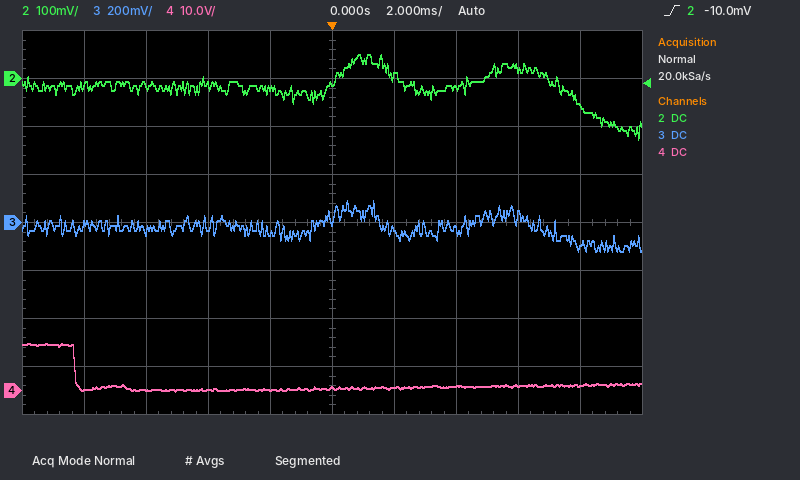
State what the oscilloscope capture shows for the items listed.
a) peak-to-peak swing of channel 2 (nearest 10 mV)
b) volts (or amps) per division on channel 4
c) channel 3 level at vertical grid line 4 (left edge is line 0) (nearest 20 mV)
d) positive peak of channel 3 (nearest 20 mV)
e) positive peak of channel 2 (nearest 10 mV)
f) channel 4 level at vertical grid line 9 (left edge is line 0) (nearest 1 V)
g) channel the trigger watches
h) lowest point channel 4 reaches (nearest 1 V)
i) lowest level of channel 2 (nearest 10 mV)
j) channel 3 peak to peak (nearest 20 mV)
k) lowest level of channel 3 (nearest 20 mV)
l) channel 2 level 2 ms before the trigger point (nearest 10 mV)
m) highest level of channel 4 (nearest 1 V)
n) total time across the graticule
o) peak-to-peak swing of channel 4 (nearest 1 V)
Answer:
180 mV
10 V
-40 mV
100 mV
50 mV
1 V
channel 2
0 V
-130 mV
220 mV
-120 mV
-20 mV
10 V
20 ms
10 V
